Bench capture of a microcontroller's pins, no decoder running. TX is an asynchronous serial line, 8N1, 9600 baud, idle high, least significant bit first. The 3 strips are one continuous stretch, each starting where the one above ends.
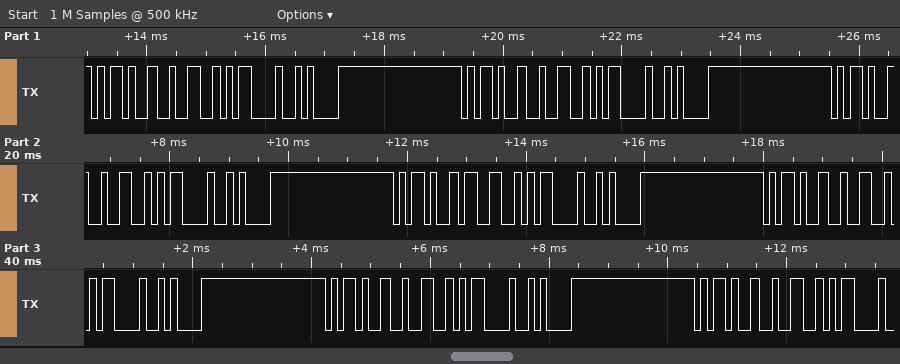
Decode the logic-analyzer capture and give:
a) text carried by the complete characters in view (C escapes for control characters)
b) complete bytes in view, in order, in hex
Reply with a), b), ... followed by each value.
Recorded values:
a) "-2\r\n-2\r\n-2\r\n-3\r\n-2\r\n-2\r\n-2\r"
b) 2D 32 0D 0A 2D 32 0D 0A 2D 32 0D 0A 2D 33 0D 0A 2D 32 0D 0A 2D 32 0D 0A 2D 32 0D
